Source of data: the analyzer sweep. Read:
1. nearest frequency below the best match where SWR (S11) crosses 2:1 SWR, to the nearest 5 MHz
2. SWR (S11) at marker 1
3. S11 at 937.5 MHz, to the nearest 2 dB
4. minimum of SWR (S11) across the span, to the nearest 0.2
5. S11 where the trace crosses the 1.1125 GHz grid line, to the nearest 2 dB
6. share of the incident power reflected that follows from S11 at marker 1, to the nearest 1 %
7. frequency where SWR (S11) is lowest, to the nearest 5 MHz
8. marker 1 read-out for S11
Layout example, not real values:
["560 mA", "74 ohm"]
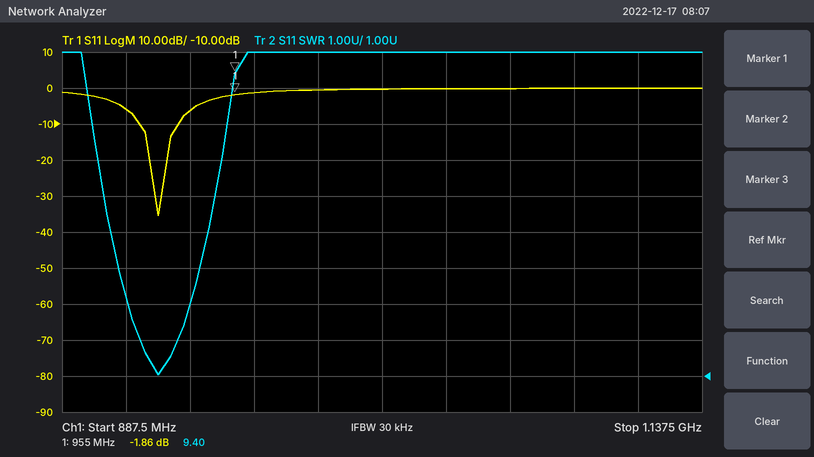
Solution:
["920 MHz", "9.40", "-6 dB", "1.0", "0 dB", "65 %", "925 MHz", "-1.86 dB"]
